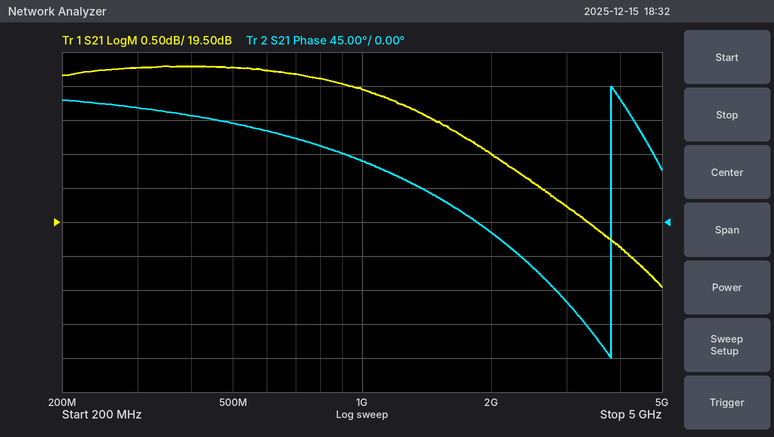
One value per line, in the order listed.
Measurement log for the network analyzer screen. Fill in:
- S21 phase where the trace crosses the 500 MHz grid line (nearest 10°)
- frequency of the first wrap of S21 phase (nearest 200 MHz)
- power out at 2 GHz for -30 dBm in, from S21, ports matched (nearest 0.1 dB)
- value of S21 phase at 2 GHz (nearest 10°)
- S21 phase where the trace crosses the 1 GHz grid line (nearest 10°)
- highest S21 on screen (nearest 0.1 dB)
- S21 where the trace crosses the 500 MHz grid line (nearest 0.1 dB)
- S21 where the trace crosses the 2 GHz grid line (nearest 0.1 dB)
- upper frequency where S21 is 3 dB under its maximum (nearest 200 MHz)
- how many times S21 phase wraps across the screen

130°
3.8 GHz
-9.5 dBm
-10°
80°
21.8 dB
21.8 dB
20.5 dB
4.6 GHz
1
